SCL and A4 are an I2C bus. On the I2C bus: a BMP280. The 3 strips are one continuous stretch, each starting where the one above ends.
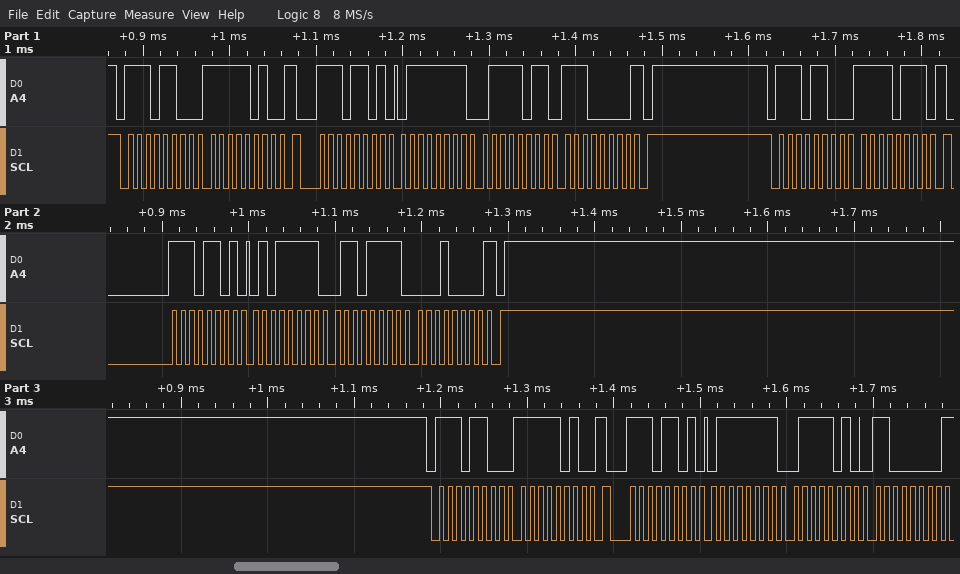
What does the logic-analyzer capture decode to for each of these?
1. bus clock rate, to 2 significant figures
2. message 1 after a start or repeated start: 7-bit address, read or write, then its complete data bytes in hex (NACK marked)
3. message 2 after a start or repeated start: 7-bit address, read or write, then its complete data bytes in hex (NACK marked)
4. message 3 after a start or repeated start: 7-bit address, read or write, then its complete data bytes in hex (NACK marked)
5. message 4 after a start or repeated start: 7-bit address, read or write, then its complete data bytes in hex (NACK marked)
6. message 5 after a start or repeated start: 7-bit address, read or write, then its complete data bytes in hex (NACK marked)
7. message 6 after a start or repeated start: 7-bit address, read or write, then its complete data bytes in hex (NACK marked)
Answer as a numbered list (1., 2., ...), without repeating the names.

1. 100 kHz
2. 0x76 write: FA
3. 0x76 read: 7F 7B E0 NACK
4. 0x76 write: F7
5. 0x76 read: 5F 6F 10 NACK
6. 0x76 write: FA
7. 0x76 read: 7F 7A C0 NACK
